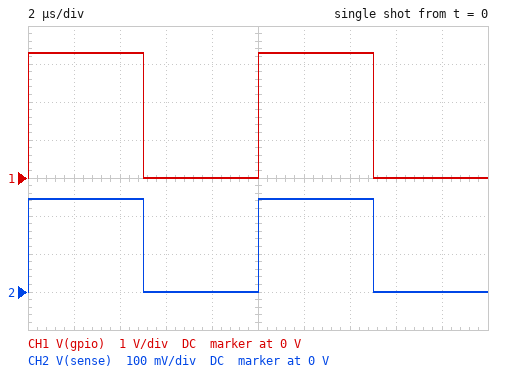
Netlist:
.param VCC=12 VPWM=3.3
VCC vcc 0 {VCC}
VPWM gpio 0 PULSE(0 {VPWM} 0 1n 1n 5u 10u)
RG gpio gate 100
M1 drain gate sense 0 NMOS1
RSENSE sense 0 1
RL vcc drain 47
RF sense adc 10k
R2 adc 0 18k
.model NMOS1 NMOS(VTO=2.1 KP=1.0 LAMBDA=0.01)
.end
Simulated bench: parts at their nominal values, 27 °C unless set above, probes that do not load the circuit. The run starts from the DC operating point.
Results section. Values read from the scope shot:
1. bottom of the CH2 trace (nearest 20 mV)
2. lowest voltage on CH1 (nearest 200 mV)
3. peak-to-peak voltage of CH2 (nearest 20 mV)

0 V
0 V
240 mV
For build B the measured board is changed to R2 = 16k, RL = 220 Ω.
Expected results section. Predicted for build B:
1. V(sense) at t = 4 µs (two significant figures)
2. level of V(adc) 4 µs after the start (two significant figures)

54 mV
33 mV
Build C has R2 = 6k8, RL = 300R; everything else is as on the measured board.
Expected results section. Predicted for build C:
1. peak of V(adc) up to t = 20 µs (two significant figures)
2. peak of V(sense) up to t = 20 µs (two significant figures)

16 mV
40 mV
